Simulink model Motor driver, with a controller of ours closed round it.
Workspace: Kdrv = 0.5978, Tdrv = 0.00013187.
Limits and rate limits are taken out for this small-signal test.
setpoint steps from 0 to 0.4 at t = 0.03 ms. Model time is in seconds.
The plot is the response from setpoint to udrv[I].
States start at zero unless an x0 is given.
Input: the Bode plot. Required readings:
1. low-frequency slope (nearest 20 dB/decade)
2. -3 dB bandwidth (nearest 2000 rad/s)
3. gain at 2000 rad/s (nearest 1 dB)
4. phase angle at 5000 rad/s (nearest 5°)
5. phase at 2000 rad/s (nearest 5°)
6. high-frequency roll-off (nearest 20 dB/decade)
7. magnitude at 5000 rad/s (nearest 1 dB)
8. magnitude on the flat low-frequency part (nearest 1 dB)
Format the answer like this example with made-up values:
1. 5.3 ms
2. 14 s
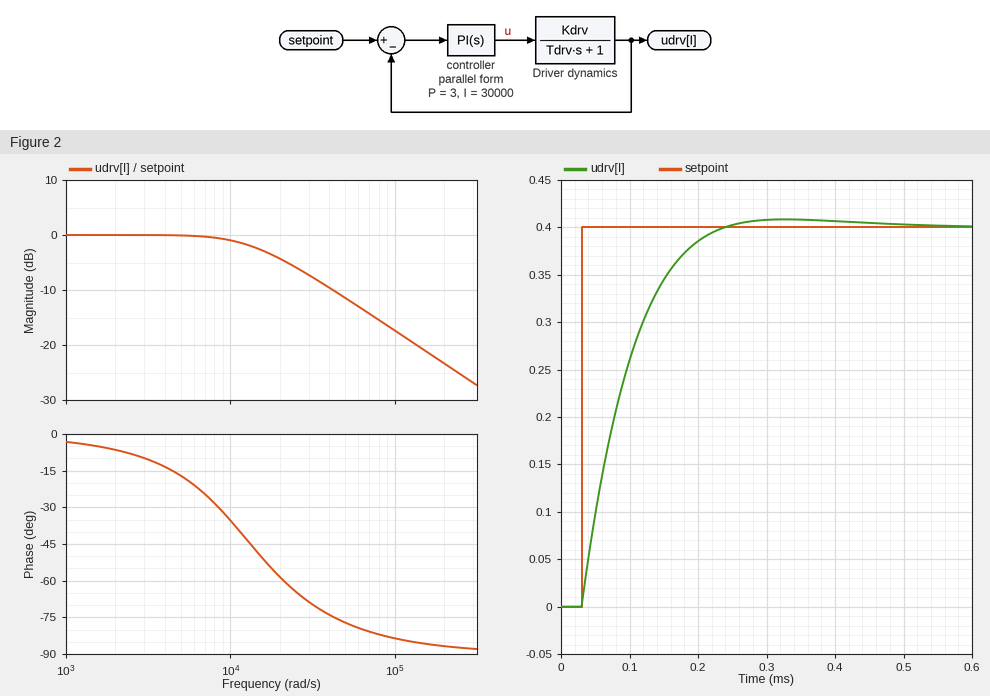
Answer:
1. 0 dB/decade
2. 16000 rad/s
3. 0 dB
4. -15°
5. -5°
6. -20 dB/decade
7. 0 dB
8. 0 dB
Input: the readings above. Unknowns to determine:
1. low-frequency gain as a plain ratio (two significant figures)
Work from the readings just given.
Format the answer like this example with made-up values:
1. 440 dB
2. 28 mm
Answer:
1. 1.0
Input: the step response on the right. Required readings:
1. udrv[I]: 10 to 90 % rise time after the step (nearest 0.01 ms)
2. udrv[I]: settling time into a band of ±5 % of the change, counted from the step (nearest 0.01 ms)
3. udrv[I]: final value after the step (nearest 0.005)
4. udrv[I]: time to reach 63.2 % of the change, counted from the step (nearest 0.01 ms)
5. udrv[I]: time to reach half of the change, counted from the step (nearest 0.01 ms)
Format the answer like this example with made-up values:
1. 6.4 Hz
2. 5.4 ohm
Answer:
1. 0.13 ms
2. 0.16 ms
3. 0.400
4. 0.07 ms
5. 0.05 ms
